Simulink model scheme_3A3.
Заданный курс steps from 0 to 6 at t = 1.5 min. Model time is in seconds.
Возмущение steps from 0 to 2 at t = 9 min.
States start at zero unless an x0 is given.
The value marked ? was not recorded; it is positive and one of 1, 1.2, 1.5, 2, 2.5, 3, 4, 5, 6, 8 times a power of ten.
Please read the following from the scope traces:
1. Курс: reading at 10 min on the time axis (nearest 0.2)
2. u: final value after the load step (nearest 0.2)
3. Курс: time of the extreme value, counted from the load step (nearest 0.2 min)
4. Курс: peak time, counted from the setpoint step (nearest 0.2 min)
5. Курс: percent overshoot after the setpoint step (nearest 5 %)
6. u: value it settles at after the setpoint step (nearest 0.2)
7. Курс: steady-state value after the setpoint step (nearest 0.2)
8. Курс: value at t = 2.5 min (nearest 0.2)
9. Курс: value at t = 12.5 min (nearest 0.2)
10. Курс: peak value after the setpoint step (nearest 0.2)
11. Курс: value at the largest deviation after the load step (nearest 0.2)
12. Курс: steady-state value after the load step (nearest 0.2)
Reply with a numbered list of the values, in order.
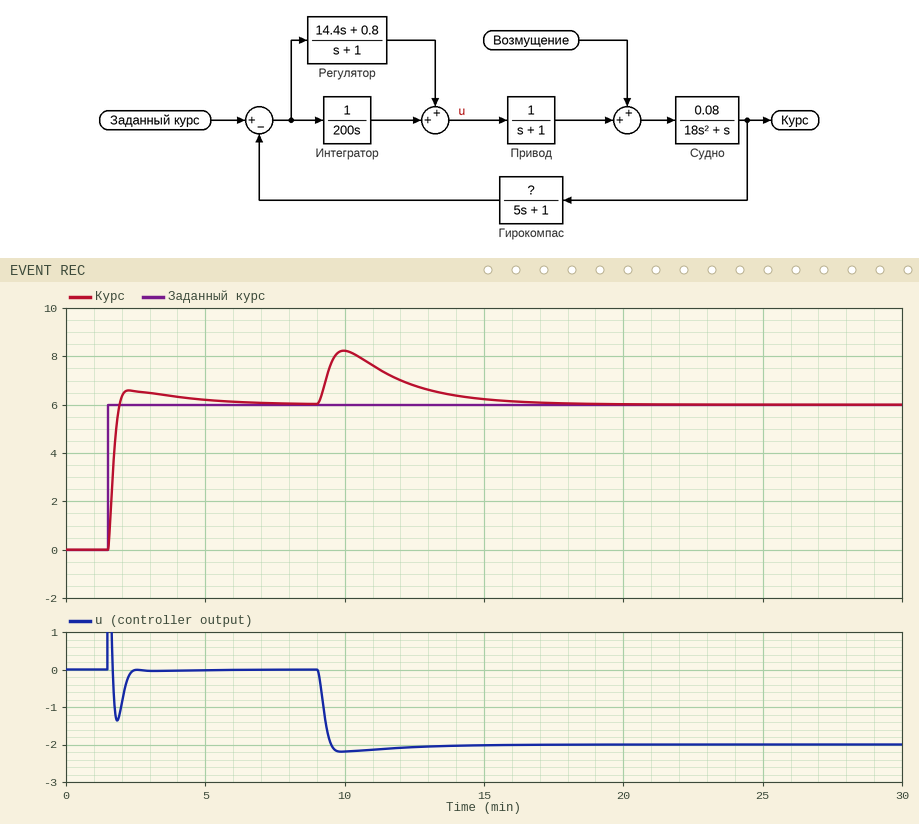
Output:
1. 8.2
2. -2.0
3. 1.0 min
4. 0.8 min
5. 10 %
6. 0.0
7. 6.0
8. 6.6
9. 6.8
10. 6.6
11. 8.2
12. 6.0
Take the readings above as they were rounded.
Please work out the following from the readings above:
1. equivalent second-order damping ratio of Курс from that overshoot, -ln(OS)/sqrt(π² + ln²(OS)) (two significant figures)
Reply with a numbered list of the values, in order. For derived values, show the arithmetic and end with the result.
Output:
1. ln(0.1) = -2.303; 2.303 / sqrt(9.870 + 5.302) = 0.59
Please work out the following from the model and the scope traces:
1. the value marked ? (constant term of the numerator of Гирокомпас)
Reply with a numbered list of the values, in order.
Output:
1. 1
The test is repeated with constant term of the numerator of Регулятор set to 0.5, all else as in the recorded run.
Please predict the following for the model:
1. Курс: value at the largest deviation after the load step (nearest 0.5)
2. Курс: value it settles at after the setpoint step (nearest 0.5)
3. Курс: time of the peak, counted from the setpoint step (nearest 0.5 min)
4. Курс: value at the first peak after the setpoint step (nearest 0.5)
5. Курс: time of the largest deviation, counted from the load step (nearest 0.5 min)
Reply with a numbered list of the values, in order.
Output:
1. 9.0
2. 6.0
3. 2.0 min
4. 7.0
5. 1.5 min
